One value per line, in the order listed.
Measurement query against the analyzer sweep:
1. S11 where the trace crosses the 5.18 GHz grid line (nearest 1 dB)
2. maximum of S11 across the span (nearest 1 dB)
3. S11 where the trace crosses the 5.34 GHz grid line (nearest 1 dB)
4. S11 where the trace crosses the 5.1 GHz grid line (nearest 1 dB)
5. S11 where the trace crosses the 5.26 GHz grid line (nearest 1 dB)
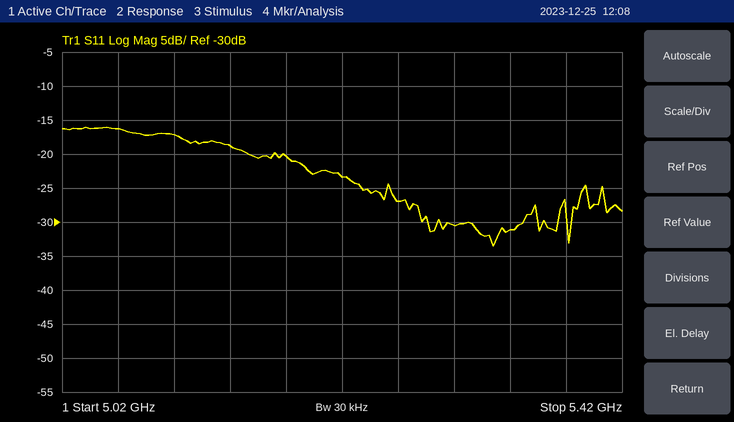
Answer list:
-20 dB
-16 dB
-31 dB
-17 dB
-27 dB
